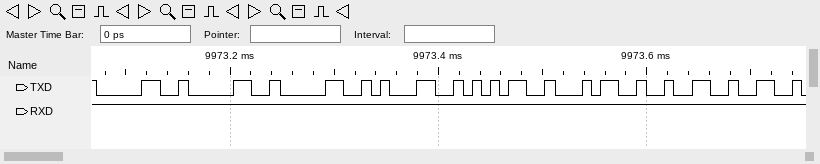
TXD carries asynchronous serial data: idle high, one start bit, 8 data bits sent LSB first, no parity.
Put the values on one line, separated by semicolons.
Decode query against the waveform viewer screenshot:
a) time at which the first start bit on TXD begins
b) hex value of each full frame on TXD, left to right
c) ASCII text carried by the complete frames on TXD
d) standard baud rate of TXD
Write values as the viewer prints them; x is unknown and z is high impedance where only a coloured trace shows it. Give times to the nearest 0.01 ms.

9973.07 ms; 30, 30, 30, 31, 35, 34, 32; "0001542"; 115200 baud
